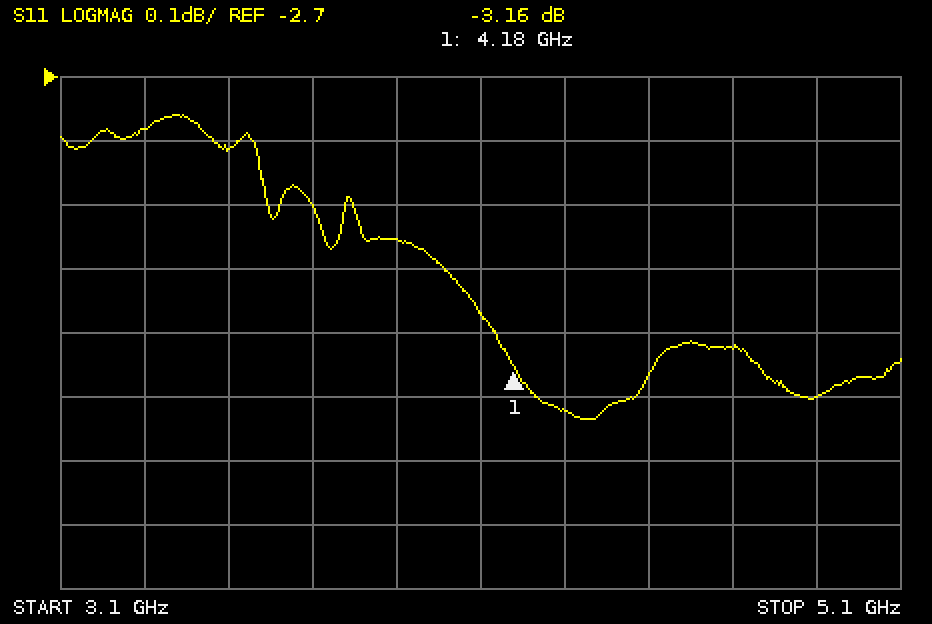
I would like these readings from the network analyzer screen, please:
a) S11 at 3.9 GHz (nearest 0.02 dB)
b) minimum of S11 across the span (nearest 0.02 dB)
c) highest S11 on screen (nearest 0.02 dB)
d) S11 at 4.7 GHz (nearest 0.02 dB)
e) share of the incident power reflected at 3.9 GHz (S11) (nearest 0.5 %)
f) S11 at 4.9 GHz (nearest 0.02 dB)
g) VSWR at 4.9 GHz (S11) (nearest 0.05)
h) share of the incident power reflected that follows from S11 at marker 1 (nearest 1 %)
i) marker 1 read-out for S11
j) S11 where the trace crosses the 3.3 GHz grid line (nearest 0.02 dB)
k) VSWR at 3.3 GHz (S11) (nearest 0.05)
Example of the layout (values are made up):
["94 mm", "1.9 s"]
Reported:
["-2.96 dB", "-3.24 dB", "-2.76 dB", "-3.12 dB", "50.5 %", "-3.20 dB", "5.50", "48 %", "-3.16 dB", "-2.78 dB", "6.30"]
